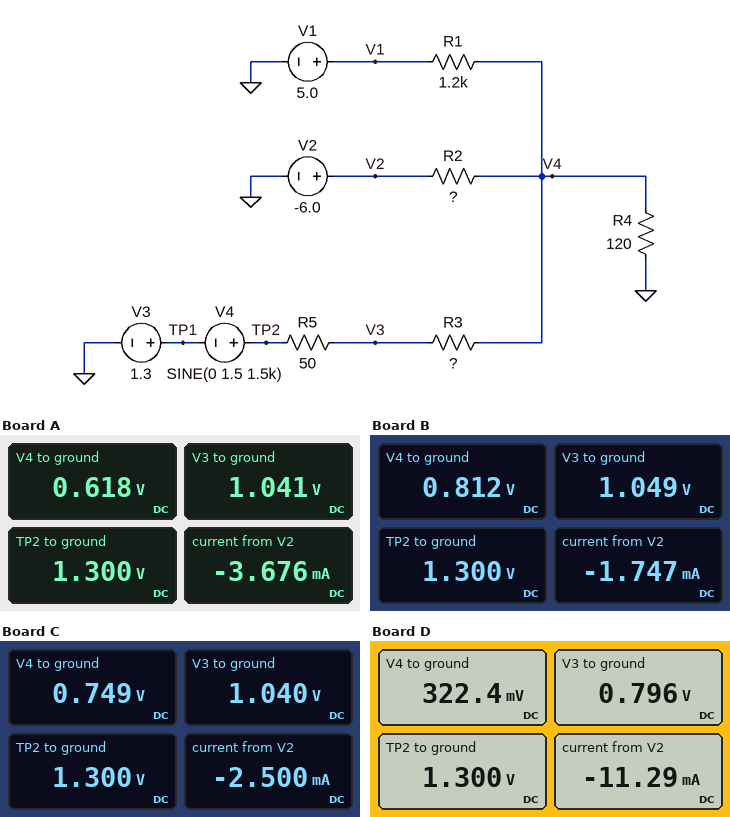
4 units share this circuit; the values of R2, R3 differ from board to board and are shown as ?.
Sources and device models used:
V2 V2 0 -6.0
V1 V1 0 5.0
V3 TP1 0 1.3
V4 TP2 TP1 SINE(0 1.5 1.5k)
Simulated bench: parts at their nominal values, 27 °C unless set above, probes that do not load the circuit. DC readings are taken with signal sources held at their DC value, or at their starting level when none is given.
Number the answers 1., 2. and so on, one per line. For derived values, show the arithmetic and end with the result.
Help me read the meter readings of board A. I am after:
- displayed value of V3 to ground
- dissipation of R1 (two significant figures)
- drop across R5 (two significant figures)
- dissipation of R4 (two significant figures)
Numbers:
1. 1.041 V
2. (5 V - 618 mV)^2 / 1.2 kΩ = 16 mW
3. 1.3 V - 1.041 V = 260 mV
4. (618 mV)^2 / 120 Ω = 3.2 mW
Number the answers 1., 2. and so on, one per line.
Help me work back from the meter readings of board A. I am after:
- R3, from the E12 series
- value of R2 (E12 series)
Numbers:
1. 82 Ω
2. 1.8 kΩ
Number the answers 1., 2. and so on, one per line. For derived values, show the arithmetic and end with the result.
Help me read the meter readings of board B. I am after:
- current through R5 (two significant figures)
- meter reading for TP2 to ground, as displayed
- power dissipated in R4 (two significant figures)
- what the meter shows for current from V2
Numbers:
1. (1.3 V - 1.049 V) / 50 Ω = 5.0 mA
2. 1.300 V
3. (812 mV)^2 / 120 Ω = 5.5 mW
4. -1.747 mA
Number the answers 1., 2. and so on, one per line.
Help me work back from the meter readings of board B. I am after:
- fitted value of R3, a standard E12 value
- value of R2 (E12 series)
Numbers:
1. 47 Ω
2. 3.9 kΩ
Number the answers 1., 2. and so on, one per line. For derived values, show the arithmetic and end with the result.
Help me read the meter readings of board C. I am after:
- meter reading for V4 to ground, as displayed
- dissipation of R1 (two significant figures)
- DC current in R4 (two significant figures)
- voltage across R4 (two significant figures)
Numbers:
1. 0.749 V
2. (5 V - 749 mV)^2 / 1.2 kΩ = 15 mW
3. (749 mV) / 120 Ω = 6.2 mA
4. 749 mV = 750 mV
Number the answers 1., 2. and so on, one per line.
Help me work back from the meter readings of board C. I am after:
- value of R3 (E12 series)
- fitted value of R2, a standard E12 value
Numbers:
1. 56 Ω
2. 2.7 kΩ
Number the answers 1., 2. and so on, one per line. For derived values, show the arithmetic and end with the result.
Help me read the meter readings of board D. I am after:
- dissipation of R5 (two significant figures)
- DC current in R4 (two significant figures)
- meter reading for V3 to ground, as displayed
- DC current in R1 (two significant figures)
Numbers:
1. (1.3 V - 796 mV)^2 / 50 Ω = 5.1 mW
2. (322.4 mV) / 120 Ω = 2.7 mA
3. 0.796 V
4. (5 V - 322.4 mV) / 1.2 kΩ = 3.9 mA
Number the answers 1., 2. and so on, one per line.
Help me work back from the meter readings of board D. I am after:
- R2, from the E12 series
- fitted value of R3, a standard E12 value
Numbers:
1. 560 Ω
2. 47 Ω
